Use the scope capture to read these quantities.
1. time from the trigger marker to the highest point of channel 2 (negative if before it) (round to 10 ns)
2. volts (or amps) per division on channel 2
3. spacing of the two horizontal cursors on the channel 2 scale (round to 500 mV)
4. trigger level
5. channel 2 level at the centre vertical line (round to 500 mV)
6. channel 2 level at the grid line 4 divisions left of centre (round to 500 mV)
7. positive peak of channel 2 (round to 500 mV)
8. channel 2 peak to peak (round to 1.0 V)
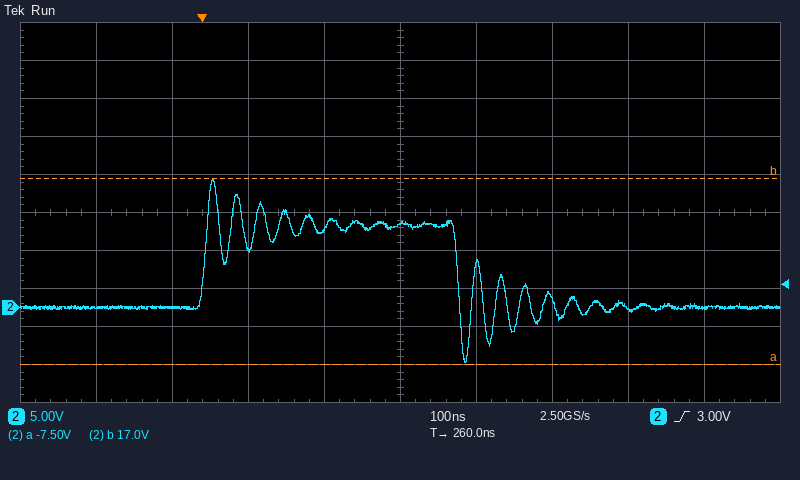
+10 ns
5 V
24.5 V
3.00 V
11.0 V
0.0 V
17.0 V
24.0 V
